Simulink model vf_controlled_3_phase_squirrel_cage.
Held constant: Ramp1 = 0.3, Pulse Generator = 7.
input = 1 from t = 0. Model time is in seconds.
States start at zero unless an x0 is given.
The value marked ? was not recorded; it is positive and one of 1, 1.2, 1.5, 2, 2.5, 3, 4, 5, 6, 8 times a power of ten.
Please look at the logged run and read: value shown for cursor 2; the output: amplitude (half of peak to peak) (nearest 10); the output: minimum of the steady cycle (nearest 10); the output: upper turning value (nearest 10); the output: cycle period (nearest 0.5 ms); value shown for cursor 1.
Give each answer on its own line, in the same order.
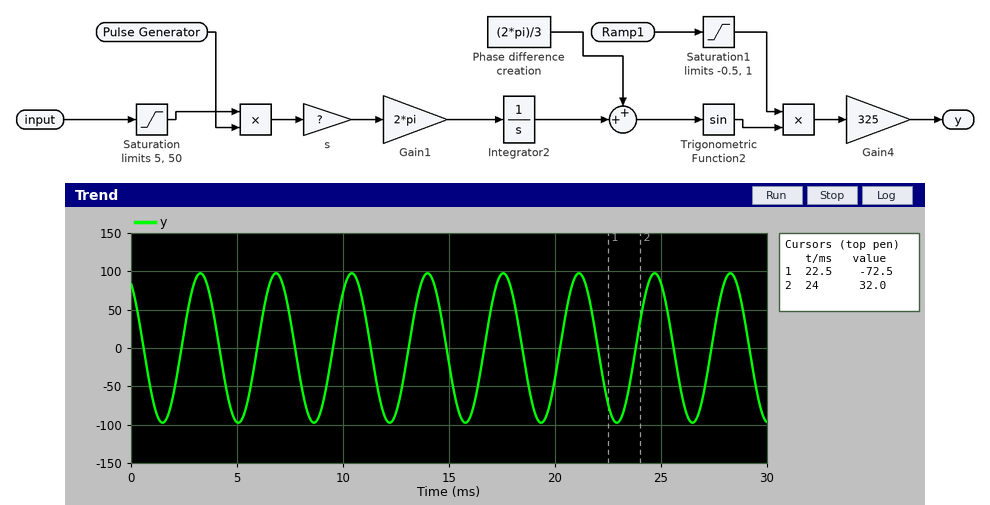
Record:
32.0
100
-100
100
3.5 ms
-72.5
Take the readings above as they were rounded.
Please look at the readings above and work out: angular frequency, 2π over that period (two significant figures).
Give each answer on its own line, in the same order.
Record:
1.8 rad/ms
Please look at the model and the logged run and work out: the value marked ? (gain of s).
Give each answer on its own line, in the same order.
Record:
8
